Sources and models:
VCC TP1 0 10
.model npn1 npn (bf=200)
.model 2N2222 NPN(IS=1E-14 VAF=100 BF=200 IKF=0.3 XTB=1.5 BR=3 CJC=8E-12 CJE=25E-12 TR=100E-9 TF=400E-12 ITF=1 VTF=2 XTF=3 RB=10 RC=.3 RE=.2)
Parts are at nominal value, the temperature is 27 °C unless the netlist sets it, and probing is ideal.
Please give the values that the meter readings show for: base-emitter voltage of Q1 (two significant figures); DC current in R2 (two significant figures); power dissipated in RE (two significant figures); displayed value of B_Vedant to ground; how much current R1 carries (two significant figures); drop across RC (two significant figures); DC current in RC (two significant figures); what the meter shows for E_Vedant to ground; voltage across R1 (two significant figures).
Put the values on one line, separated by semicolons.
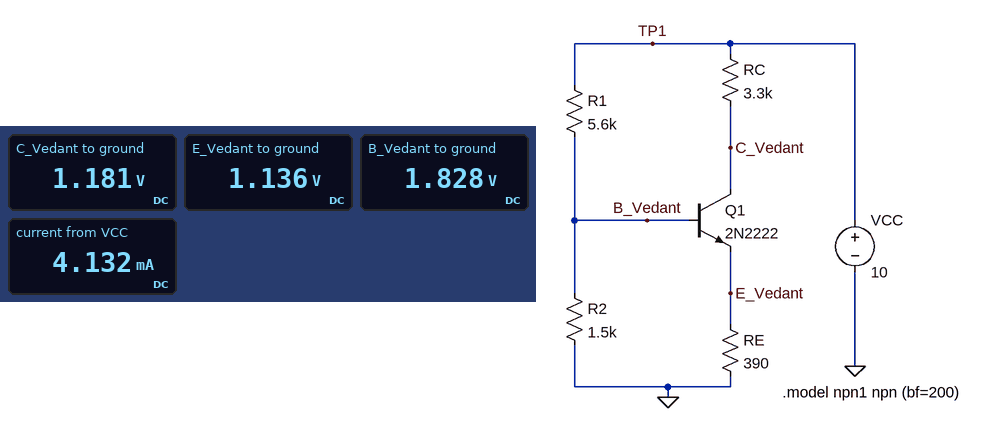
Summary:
690 mV; 1.2 mA; 3.3 mW; 1.828 V; 1.5 mA; 8.8 V; 2.7 mA; 1.136 V; 8.2 V
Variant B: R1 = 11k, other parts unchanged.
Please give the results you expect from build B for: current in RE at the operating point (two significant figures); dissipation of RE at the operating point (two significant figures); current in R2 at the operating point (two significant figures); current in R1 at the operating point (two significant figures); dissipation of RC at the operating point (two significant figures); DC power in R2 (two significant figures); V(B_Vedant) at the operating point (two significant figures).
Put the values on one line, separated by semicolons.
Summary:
1.4 mA; 720 µW; 790 µA; 800 µA; 6.0 mW; 950 µW; 1.2 V
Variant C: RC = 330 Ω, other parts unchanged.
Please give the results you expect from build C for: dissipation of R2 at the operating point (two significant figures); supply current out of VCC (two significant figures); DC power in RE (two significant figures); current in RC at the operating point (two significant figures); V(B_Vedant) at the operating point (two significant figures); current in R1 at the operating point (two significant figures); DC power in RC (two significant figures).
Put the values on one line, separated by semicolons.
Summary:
2.9 mW; 5.0 mA; 5.1 mW; 3.6 mA; 2.1 V; 1.4 mA; 4.2 mW
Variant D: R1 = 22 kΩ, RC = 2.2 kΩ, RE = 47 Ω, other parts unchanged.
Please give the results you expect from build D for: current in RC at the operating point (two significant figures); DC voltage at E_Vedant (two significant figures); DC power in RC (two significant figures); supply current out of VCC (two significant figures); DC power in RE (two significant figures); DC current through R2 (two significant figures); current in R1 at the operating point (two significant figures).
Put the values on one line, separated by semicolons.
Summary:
300 µA; 14 mV; 200 µW; 730 µA; 4.3 µW; 420 µA; 430 µA
